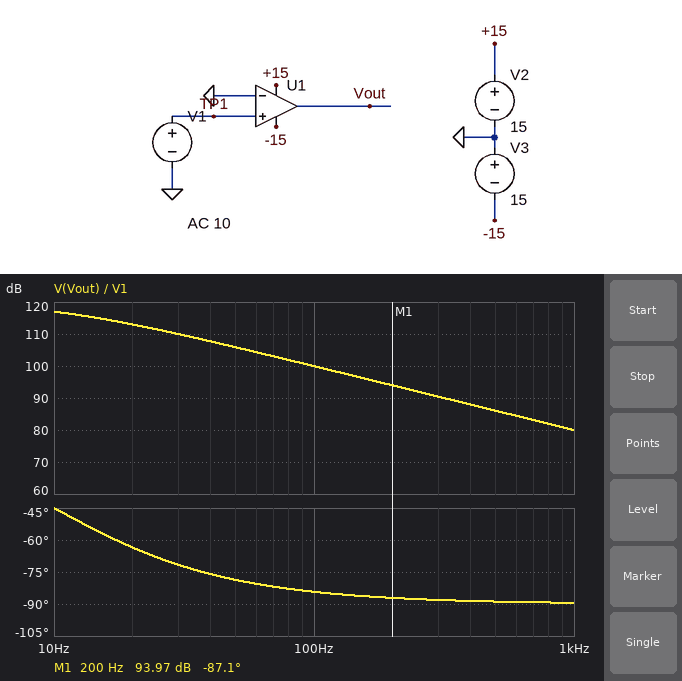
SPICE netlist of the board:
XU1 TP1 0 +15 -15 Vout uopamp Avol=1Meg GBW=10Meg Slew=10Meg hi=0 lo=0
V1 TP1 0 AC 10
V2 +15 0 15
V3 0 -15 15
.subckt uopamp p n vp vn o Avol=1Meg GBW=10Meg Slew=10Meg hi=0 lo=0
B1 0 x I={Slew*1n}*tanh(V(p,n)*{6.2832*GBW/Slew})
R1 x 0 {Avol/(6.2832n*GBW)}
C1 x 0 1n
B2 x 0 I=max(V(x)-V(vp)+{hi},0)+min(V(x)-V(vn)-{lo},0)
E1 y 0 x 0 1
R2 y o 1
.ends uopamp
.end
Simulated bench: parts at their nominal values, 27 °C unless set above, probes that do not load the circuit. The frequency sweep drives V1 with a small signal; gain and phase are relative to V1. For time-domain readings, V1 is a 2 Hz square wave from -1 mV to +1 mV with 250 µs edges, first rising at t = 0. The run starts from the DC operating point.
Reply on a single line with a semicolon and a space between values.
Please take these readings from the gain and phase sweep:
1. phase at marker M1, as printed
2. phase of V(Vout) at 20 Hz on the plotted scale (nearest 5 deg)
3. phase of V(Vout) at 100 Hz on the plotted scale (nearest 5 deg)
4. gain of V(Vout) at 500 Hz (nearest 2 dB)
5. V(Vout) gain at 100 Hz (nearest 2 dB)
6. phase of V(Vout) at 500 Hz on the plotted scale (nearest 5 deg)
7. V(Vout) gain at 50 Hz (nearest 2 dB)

-87.1 deg; -65 deg; -85 deg; 86 dB; 100 dB; -90 deg; 106 dB
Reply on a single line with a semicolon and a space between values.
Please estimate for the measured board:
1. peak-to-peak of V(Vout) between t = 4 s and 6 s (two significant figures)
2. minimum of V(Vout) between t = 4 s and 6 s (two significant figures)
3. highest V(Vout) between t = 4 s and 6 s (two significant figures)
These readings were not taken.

30 V; -15 V; 15 V
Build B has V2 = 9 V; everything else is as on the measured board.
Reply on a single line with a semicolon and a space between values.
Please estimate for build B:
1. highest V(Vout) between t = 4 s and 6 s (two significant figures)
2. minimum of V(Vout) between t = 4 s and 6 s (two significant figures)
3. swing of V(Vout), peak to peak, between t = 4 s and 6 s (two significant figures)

9.0 V; -15 V; 24 V
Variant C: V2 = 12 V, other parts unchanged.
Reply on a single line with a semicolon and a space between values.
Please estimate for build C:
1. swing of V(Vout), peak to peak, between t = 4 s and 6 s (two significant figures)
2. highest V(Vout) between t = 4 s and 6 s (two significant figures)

27 V; 12 V
